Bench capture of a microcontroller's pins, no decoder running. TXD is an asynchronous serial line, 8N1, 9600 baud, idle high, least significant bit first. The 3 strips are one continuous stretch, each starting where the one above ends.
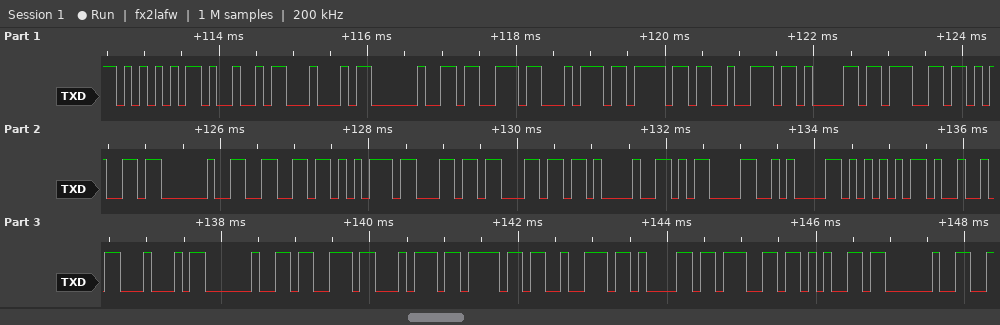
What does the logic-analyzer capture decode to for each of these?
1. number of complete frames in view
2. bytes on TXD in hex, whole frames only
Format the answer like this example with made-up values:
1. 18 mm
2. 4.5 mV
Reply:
1. 31
2. 55 49 44 20 73 74 6F 72 61 67 65 20 66 75 6C 6C 21 0D 0A 55 49 44 20 73 74 6F 72 61 67 65 20
